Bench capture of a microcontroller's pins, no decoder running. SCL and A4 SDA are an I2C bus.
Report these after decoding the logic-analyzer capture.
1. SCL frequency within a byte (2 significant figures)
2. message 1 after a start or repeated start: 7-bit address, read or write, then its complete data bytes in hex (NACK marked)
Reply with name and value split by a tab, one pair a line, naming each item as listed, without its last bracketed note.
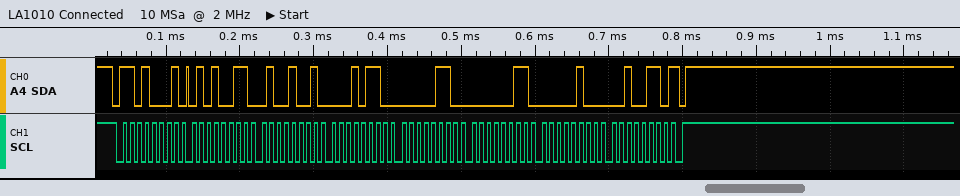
SCL frequency within a byte	100 kHz
message 1 after a start or repeated start: 7-bit address, read or write, then its complete data bytes in hex	0x68 read: 53 49 16 06 03 04 26 NACK
